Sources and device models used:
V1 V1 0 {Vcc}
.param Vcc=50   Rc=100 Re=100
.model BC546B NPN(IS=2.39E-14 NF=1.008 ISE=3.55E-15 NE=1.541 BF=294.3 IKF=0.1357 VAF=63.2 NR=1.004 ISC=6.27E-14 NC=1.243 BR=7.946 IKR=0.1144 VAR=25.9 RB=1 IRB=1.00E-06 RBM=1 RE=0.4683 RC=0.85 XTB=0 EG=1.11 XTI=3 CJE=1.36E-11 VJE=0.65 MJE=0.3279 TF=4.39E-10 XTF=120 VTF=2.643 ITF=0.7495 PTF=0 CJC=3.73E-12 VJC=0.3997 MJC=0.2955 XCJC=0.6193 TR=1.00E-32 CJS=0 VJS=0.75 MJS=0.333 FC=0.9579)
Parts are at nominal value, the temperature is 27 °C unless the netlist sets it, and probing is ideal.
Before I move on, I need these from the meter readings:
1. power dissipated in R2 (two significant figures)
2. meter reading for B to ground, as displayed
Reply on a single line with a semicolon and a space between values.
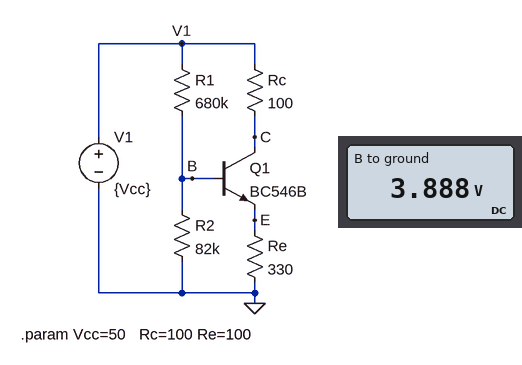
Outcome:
180 µW; 3.888 V
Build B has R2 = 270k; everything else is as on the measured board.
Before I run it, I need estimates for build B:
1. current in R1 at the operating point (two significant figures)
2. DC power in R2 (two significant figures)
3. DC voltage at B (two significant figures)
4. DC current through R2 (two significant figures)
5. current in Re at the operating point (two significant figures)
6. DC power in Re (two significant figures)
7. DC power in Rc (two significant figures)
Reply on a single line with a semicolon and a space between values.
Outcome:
64 µA; 160 µW; 6.5 V; 24 µA; 18 mA; 100 mW; 31 mW
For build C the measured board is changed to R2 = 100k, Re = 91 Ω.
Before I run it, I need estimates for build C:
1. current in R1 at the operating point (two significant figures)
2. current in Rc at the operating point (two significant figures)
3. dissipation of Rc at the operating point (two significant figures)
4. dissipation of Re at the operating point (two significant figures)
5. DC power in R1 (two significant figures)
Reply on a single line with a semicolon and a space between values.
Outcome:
70 µA; 20 mA; 41 mW; 37 mW; 3.3 mW
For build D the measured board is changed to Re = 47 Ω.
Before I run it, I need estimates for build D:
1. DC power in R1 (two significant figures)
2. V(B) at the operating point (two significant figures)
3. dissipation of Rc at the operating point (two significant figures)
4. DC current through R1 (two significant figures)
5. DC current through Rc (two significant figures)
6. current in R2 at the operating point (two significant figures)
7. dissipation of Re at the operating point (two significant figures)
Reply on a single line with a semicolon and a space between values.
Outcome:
3.4 mW; 1.8 V; 50 mW; 71 µA; 22 mA; 22 µA; 24 mW
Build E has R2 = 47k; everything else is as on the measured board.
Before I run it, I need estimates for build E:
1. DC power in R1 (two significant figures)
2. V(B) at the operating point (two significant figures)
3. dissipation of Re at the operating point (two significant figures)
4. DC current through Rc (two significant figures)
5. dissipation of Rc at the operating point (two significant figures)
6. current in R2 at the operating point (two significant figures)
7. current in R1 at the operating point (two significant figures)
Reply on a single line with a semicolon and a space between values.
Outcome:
3.3 mW; 2.7 V; 12 mW; 6.1 mA; 3.7 mW; 57 µA; 70 µA
